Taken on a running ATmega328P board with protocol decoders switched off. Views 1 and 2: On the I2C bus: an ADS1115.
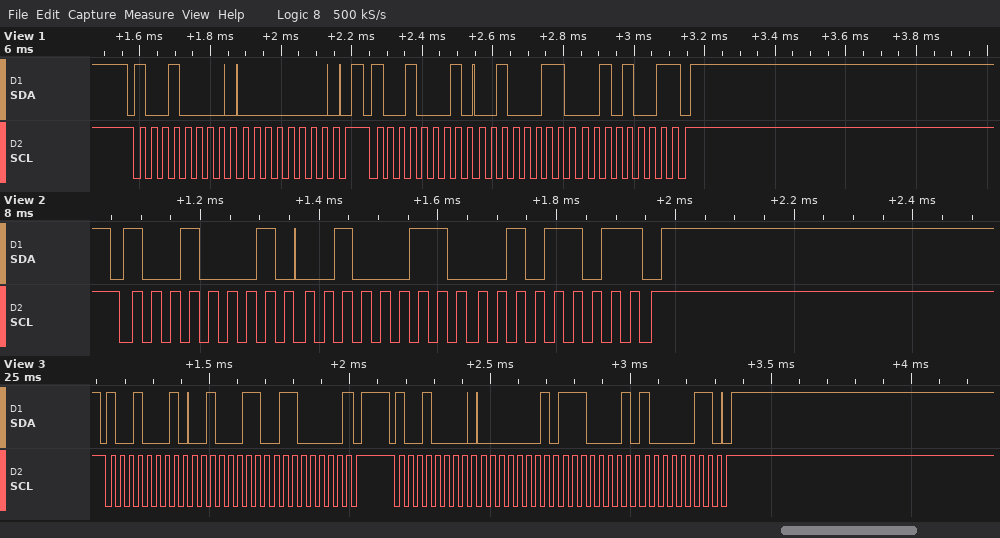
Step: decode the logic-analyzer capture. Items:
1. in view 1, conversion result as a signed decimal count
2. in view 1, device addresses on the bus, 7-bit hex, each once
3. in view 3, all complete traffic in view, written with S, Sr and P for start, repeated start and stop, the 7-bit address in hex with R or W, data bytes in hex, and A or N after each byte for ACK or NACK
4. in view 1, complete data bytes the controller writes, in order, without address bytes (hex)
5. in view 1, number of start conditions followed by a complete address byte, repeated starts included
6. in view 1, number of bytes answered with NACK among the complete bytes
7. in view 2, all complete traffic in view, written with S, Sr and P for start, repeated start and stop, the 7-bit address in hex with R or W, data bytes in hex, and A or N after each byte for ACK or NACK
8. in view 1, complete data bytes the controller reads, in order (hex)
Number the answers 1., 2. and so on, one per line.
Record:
1. 9001
2. 0x48
3. S 48R A 23 A 60 N P S 48W A 01 A E1 A 83 A P
4. 00
5. 2
6. 1
7. S 48R A 23 A 2D N P
8. 23 29
